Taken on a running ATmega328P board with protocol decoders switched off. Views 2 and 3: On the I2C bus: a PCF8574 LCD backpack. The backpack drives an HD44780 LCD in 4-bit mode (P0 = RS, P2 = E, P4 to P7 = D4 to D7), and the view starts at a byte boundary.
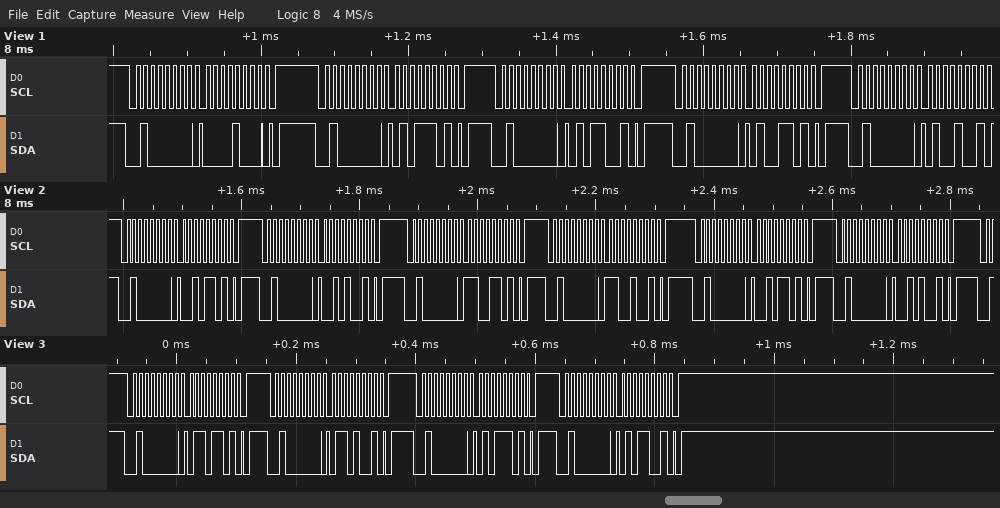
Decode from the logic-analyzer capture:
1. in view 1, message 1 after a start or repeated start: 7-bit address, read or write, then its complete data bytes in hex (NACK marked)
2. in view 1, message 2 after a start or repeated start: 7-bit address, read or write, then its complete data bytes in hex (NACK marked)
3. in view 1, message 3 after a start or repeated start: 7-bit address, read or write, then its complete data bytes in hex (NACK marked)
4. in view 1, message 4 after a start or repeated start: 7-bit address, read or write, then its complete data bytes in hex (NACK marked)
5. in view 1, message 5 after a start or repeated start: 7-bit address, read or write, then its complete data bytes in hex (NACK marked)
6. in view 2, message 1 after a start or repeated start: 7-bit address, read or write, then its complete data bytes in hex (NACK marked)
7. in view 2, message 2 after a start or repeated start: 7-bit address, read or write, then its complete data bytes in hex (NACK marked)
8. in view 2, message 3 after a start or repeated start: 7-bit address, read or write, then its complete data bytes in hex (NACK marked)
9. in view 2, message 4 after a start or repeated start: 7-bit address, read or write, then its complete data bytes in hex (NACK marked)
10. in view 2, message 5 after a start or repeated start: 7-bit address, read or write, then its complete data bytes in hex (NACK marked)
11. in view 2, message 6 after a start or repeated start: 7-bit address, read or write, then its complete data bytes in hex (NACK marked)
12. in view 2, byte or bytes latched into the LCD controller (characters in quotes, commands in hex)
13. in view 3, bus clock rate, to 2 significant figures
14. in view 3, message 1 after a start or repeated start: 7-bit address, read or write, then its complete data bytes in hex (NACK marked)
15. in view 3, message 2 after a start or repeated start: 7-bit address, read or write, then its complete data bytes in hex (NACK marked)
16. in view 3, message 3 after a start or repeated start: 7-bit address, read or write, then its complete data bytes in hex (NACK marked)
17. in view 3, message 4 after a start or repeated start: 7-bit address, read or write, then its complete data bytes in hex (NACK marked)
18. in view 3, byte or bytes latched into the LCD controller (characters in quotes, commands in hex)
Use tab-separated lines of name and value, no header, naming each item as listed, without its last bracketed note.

in view 1, message 1 after a start or repeated start: 7-bit address, read or write, then its complete data bytes in hex	0x20 write: 08
in view 1, message 2 after a start or repeated start: 7-bit address, read or write, then its complete data bytes in hex	0x20 write: 5D
in view 1, message 3 after a start or repeated start: 7-bit address, read or write, then its complete data bytes in hex	0x20 write: 59
in view 1, message 4 after a start or repeated start: 7-bit address, read or write, then its complete data bytes in hex	0x20 write: 4D
in view 1, message 5 after a start or repeated start: 7-bit address, read or write, then its complete data bytes in hex	0x20 write: 49
in view 2, message 1 after a start or repeated start: 7-bit address, read or write, then its complete data bytes in hex	0x20 write: 2D
in view 2, message 2 after a start or repeated start: 7-bit address, read or write, then its complete data bytes in hex	0x20 write: 29
in view 2, message 3 after a start or repeated start: 7-bit address, read or write, then its complete data bytes in hex	0x20 write: CD
in view 2, message 4 after a start or repeated start: 7-bit address, read or write, then its complete data bytes in hex	0x20 write: C9
in view 2, message 5 after a start or repeated start: 7-bit address, read or write, then its complete data bytes in hex	0x20 write: 2D
in view 2, message 6 after a start or repeated start: 7-bit address, read or write, then its complete data bytes in hex	0x20 write: 29
in view 2, byte or bytes latched into the LCD controller	','
in view 3, bus clock rate, to 2 significant figures	100 kHz
in view 3, message 1 after a start or repeated start: 7-bit address, read or write, then its complete data bytes in hex	0x20 write: 6D
in view 3, message 2 after a start or repeated start: 7-bit address, read or write, then its complete data bytes in hex	0x20 write: 69
in view 3, message 3 after a start or repeated start: 7-bit address, read or write, then its complete data bytes in hex	0x20 write: 5D
in view 3, message 4 after a start or repeated start: 7-bit address, read or write, then its complete data bytes in hex	0x20 write: 59
in view 3, byte or bytes latched into the LCD controller	'e'
